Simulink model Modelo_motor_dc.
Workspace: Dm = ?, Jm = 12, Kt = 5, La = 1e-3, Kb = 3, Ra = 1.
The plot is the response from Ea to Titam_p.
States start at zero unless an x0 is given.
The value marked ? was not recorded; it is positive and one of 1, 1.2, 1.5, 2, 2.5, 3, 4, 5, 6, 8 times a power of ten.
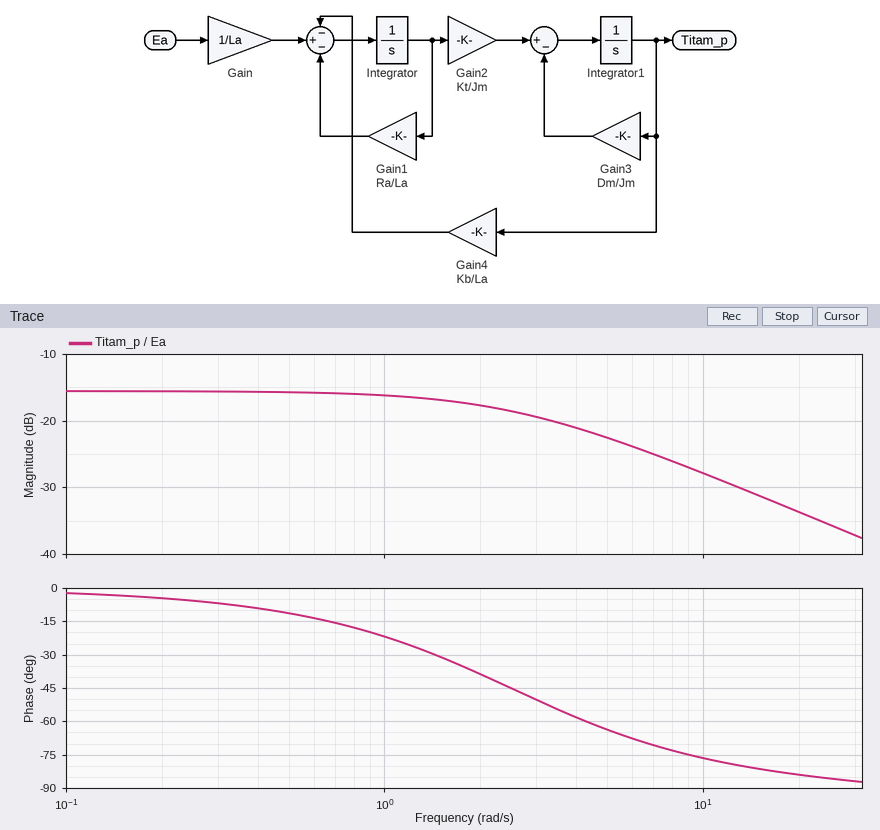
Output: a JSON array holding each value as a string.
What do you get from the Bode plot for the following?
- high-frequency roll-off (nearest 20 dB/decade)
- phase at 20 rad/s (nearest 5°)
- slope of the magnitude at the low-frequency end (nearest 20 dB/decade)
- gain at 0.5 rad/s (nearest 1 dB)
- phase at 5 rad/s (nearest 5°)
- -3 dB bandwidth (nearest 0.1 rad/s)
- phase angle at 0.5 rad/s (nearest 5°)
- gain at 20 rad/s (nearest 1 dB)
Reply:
["-20 dB/decade", "-85°", "0 dB/decade", "-16 dB", "-65°", "2.5 rad/s", "-10°", "-34 dB"]
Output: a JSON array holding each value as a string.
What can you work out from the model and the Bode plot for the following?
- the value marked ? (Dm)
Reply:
["15"]
